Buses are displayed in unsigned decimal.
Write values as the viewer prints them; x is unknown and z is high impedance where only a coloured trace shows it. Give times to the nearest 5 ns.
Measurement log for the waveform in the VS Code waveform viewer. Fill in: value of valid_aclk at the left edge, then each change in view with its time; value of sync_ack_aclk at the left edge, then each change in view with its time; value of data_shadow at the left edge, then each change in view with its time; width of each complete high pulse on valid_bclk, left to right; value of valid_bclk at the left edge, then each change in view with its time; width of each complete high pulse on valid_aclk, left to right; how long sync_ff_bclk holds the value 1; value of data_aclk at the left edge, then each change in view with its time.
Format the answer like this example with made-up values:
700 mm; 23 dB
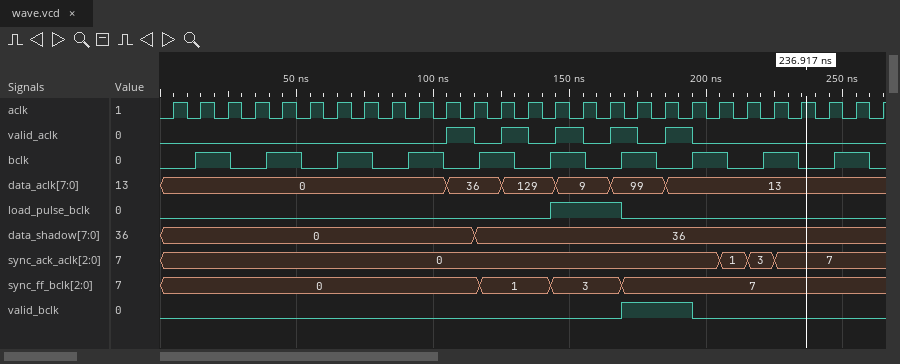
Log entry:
0, 1 at 105 ns, 0 at 115 ns, 1 at 125 ns, 0 at 135 ns, 1 at 145 ns, 0 at 155 ns, 1 at 165 ns, 0 at 175 ns, 1 at 185 ns, 0 at 195 ns; 0, 1 at 205 ns, 3 at 215 ns, 7 at 225 ns; 0, 36 at 115 ns; 25 ns; 0, 1 at 170 ns, 0 at 195 ns; 10 ns, 10 ns, 10 ns, 10 ns, 10 ns; 25 ns; 0, 36 at 105 ns, 129 at 125 ns, 9 at 145 ns, 99 at 165 ns, 13 at 185 ns
